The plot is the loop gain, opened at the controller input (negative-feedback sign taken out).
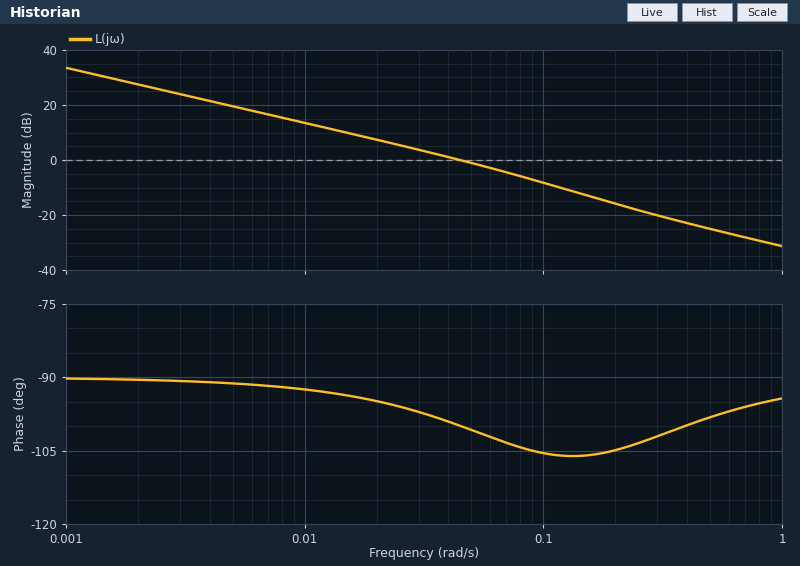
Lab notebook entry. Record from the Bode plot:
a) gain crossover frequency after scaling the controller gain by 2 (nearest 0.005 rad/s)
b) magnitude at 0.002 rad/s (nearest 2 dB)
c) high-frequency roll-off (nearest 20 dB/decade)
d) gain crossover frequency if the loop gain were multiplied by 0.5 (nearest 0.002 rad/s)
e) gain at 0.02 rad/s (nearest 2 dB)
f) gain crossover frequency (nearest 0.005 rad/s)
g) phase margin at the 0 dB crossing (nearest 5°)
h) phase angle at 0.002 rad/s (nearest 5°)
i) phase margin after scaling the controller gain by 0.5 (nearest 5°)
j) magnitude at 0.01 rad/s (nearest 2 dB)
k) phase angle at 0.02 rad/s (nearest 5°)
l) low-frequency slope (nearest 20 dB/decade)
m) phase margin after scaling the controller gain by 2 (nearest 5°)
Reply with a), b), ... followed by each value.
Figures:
a) 0.080 rad/s
b) 28 dB
c) -20 dB/decade
d) 0.024 rad/s
e) 8 dB
f) 0.045 rad/s
g) 80°
h) -90°
i) 85°
j) 14 dB
k) -95°
l) -20 dB/decade
m) 75°
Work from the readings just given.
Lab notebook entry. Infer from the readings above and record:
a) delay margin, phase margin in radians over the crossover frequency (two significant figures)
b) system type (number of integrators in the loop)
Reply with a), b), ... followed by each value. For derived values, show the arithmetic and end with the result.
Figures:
a) 80 × π / 180 / 0.045 = 31 s
b) 1
